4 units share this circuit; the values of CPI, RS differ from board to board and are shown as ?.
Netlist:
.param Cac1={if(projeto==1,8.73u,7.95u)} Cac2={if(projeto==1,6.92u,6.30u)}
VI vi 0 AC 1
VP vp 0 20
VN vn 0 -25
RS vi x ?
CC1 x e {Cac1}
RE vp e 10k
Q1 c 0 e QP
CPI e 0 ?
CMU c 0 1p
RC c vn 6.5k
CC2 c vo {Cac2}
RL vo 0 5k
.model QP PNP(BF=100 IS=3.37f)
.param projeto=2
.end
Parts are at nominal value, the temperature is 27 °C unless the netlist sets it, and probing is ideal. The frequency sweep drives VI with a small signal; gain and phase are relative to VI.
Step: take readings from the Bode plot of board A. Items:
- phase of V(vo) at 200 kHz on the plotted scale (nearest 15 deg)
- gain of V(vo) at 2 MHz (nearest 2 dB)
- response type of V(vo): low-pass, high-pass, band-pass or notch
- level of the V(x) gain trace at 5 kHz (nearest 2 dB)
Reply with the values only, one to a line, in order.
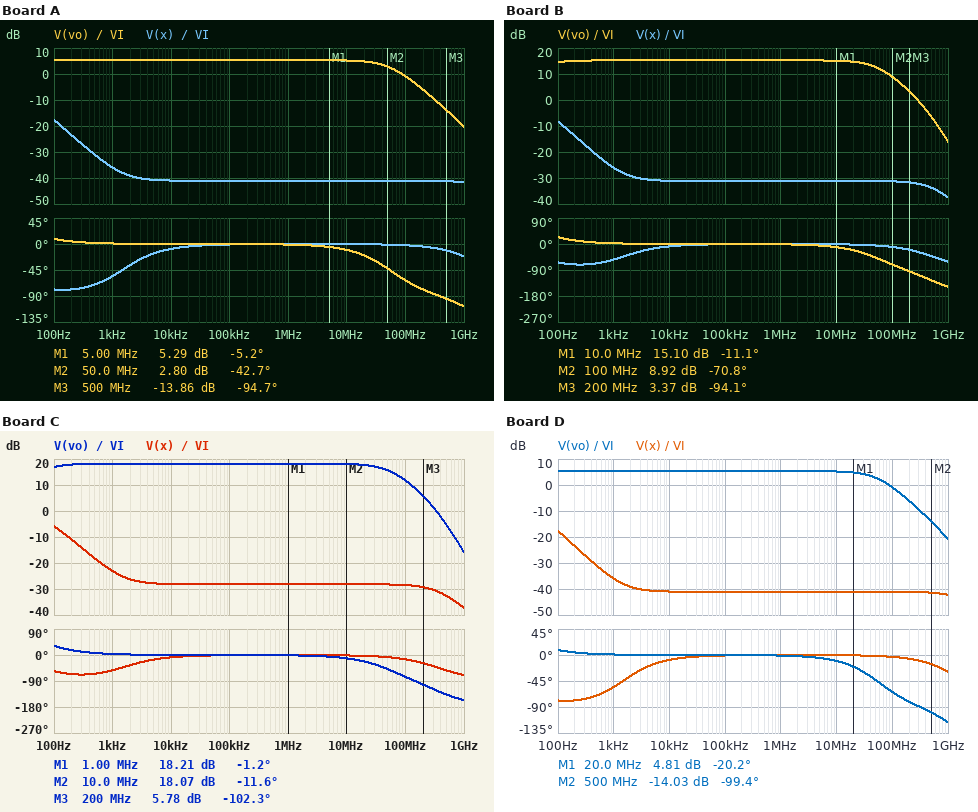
0 deg
6 dB
low-pass
-40 dB
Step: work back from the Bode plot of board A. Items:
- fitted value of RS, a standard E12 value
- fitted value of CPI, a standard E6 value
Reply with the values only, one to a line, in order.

1.5 kΩ
4.7 pF
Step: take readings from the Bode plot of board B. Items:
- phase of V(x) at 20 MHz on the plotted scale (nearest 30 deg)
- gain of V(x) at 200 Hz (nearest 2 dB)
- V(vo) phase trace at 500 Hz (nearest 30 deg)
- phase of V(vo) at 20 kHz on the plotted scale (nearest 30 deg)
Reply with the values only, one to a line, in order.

0 deg
-14 dB
0 deg
0 deg
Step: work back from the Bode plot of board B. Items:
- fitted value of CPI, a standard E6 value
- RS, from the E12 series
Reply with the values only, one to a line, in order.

22 pF
470 Ω
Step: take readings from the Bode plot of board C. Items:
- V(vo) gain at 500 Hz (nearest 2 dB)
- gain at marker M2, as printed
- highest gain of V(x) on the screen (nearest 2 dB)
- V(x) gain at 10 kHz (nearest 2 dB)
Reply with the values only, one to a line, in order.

18 dB
18.07 dB
-6 dB
-28 dB
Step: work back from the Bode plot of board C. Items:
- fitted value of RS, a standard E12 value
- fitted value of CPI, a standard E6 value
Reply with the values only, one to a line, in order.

330 Ω
33 pF
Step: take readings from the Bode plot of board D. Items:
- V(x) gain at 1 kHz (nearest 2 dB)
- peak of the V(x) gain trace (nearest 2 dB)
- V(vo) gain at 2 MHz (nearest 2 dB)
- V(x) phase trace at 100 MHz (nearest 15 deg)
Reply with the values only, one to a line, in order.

-36 dB
-18 dB
6 dB
0 deg
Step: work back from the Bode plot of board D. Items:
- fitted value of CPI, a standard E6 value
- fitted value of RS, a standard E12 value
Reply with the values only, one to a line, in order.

6.8 pF
1.5 kΩ
